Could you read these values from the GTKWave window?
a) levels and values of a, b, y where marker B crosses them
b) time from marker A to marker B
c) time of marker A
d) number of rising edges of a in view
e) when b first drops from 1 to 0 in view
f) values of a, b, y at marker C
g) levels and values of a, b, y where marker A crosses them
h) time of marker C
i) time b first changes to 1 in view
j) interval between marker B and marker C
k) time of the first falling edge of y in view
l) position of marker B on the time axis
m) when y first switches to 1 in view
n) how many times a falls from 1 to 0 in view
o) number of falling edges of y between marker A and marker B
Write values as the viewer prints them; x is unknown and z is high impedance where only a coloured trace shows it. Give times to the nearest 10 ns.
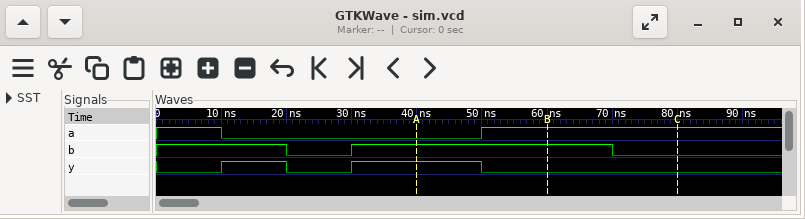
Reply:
a=1, b=1, y=0
20 ns
40 ns
1
20 ns
a=1, b=0, y=0
a=0, b=1, y=1
80 ns
30 ns
20 ns
20 ns
60 ns
10 ns
1
1
